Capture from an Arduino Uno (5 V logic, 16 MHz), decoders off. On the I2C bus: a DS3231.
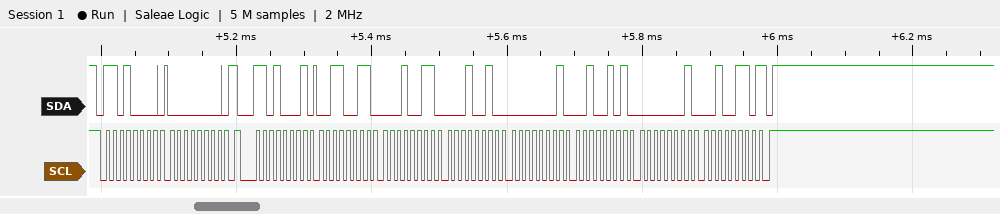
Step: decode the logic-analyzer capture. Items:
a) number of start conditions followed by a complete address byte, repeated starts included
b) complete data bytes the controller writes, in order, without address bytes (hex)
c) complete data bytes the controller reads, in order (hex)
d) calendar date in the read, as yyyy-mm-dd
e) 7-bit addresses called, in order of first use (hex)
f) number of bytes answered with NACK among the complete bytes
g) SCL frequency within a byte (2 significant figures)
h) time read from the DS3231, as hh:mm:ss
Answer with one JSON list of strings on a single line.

["2", "00", "33 13 12 01 25 01 26", "2026-01-25", "0x68", "1", "100 kHz", "12:13:33"]
